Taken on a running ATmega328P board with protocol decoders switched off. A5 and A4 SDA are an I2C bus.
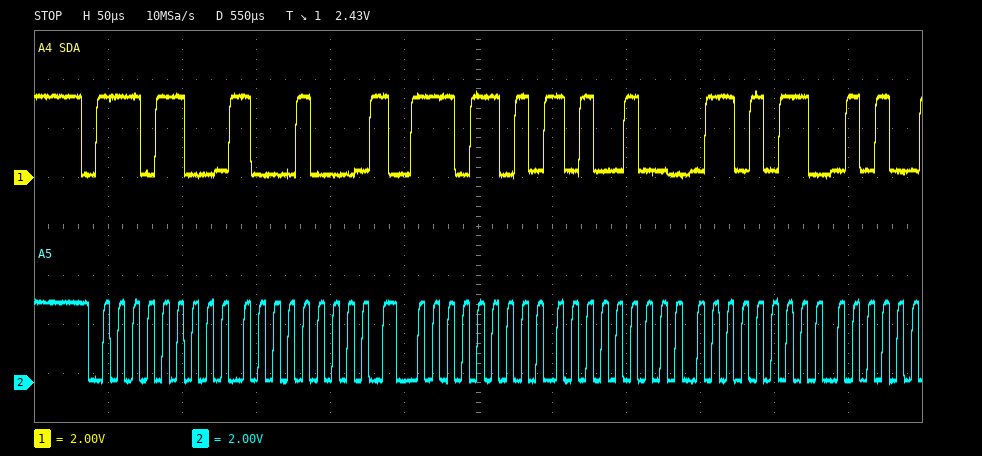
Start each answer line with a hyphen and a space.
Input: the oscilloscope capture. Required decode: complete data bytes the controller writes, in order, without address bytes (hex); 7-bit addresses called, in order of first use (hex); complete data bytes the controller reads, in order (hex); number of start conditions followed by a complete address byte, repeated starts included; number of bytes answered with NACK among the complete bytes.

- 88
- 0x76
- A4 6B
- 2
- 0
